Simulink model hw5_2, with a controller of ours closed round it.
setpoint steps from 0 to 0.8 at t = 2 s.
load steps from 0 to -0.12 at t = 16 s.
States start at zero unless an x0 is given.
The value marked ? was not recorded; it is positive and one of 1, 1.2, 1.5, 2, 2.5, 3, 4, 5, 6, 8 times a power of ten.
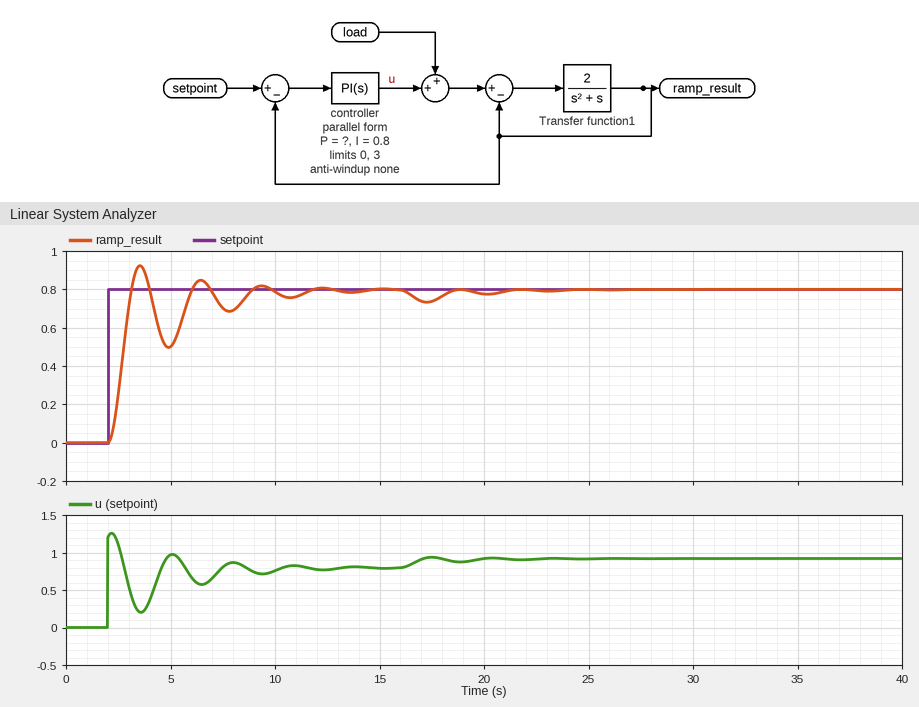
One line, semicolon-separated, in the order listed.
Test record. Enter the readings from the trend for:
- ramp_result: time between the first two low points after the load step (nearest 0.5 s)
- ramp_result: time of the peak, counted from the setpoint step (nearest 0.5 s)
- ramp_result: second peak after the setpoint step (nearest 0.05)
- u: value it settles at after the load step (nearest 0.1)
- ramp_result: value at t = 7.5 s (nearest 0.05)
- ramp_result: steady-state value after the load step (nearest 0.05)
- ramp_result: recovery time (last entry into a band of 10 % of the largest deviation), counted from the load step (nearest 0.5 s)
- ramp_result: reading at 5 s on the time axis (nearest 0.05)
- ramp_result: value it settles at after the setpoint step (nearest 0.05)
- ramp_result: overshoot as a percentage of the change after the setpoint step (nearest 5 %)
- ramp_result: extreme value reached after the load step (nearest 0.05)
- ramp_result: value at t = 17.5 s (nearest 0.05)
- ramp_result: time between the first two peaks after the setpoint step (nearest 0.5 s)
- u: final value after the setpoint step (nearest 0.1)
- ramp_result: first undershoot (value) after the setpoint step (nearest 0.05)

3.0 s; 1.5 s; 0.85; 0.9; 0.70; 0.80; 7.5 s; 0.50; 0.80; 15 %; 0.75; 0.75; 3.0 s; 0.8; 0.50
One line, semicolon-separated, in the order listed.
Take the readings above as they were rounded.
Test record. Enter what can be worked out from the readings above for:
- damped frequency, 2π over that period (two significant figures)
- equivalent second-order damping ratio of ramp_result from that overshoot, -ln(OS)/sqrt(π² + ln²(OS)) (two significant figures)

2.1 rad/s; 0.52
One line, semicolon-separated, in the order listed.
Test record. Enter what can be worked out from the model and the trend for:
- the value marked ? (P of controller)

1.5
